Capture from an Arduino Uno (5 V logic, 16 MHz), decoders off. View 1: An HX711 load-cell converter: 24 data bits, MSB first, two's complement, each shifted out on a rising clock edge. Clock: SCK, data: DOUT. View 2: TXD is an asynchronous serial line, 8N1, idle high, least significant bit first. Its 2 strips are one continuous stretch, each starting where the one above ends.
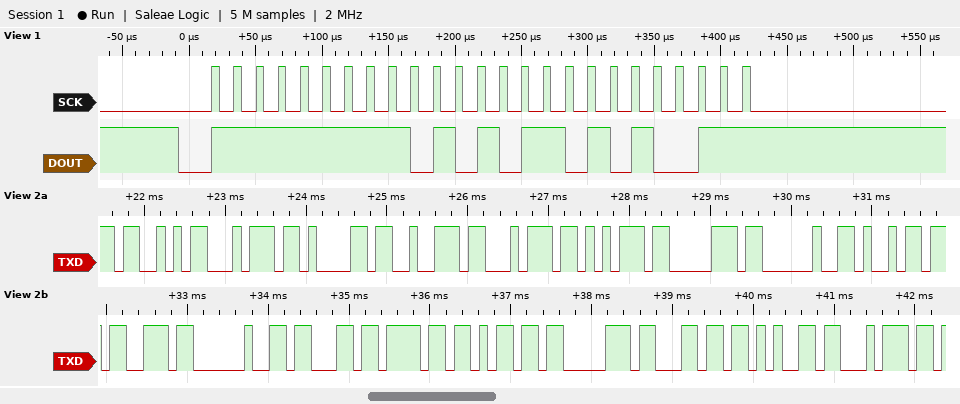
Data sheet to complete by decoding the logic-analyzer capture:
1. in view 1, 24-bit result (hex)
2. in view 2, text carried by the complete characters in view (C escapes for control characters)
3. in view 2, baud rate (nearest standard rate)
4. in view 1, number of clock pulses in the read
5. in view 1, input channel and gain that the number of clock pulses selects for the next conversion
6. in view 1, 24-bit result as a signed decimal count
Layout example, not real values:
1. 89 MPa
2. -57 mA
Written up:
1. 0xFFAB53
2. "Startup is complet"
3. 9600 baud
4. 25
5. channel A, gain 128
6. -21677
